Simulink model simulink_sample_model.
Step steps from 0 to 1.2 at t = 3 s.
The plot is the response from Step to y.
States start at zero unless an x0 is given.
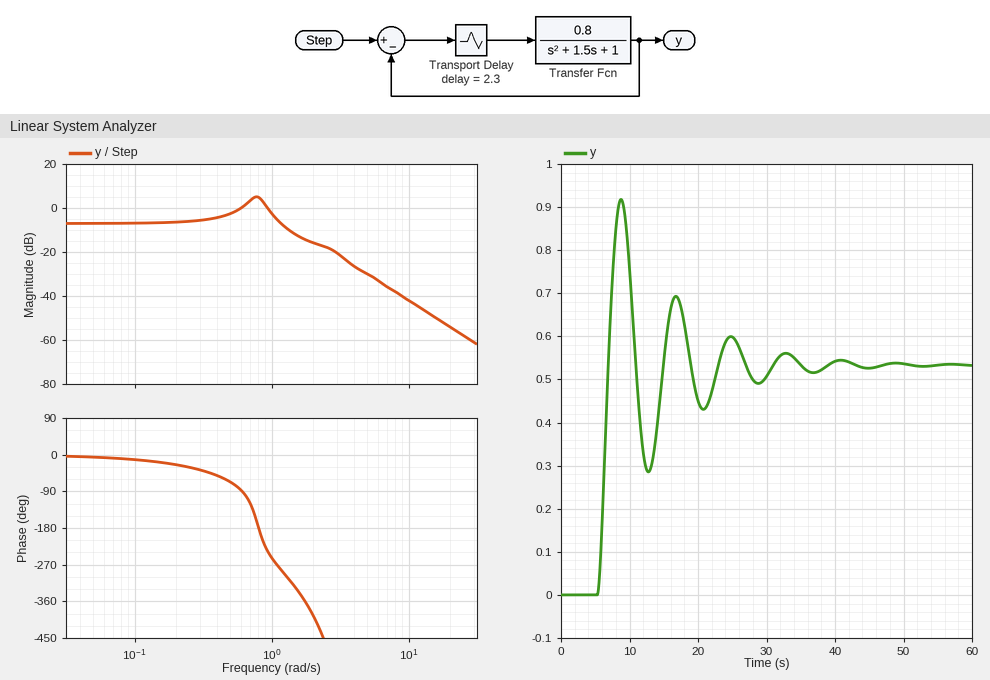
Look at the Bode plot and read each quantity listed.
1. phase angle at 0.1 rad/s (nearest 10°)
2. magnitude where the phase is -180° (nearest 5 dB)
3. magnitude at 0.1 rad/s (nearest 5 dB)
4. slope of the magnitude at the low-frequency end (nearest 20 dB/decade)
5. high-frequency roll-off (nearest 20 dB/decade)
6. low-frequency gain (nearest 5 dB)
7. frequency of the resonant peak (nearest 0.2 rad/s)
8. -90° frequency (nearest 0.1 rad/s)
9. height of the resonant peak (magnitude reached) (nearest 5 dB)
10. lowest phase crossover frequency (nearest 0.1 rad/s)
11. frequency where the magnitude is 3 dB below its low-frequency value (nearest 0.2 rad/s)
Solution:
-10°
5 dB
-5 dB
0 dB/decade
-40 dB/decade
-5 dB
0.8 rad/s
0.6 rad/s
5 dB
0.8 rad/s
1.4 rad/s
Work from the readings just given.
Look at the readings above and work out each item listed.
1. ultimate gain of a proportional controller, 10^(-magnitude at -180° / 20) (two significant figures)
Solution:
0.56
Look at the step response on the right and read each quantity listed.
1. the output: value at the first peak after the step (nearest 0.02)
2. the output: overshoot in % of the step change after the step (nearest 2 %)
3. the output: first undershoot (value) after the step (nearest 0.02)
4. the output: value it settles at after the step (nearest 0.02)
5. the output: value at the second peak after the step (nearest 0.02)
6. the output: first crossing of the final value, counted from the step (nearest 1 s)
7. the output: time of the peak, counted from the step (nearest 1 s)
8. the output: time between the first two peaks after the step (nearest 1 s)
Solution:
0.92
72 %
0.28
0.54
0.70
4 s
6 s
8 s
